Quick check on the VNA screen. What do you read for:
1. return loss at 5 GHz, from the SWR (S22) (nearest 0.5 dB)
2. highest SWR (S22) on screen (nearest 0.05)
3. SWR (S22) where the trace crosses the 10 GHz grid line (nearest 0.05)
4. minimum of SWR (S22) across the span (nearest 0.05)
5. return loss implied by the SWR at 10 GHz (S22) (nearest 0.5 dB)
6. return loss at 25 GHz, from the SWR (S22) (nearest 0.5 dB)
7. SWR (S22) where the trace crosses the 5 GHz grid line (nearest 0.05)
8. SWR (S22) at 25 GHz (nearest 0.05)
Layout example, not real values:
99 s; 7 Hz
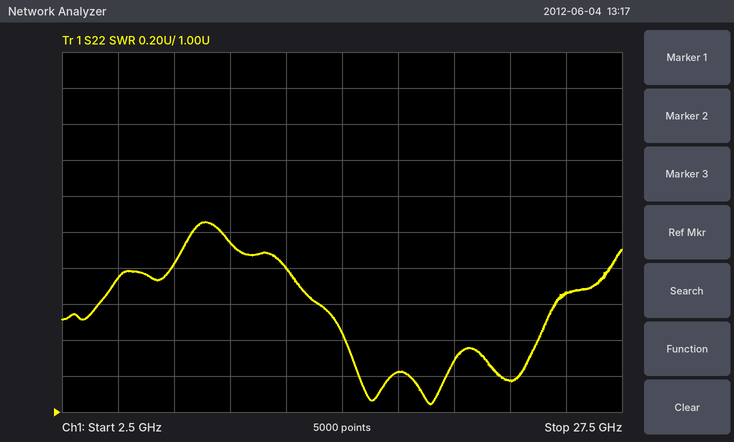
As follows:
11.5 dB; 2.05; 1.95; 1.05; 10.0 dB; 12.0 dB; 1.75; 1.65
